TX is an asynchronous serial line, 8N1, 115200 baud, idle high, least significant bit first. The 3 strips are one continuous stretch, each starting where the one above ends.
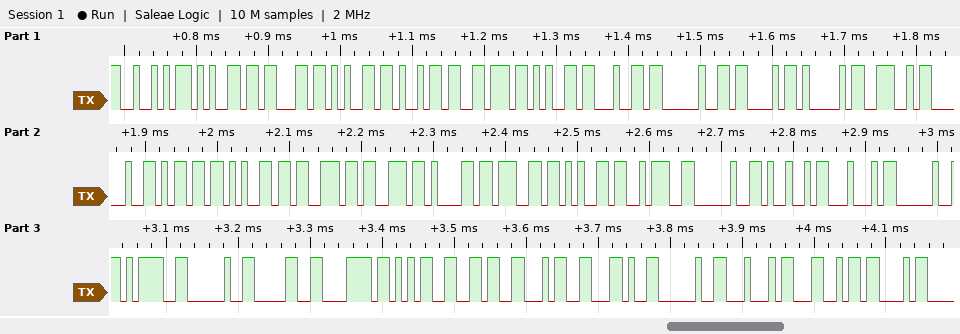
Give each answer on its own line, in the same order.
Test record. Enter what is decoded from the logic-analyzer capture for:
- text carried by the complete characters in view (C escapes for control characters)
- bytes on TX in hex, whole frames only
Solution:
"Received CAN message: ID = 0x564, DLC"
52 65 63 65 69 76 65 64 20 43 41 4E 20 6D 65 73 73 61 67 65 3A 20 49 44 20 3D 20 30 78 35 36 34 2C 20 44 4C 43
